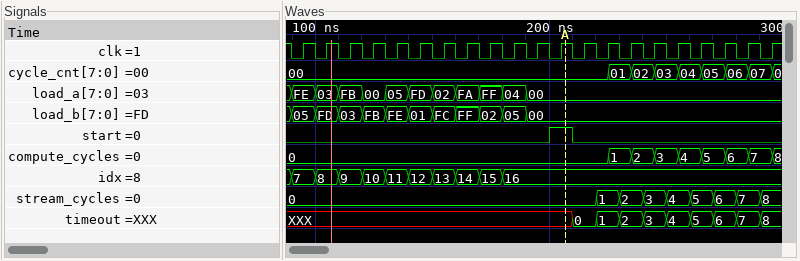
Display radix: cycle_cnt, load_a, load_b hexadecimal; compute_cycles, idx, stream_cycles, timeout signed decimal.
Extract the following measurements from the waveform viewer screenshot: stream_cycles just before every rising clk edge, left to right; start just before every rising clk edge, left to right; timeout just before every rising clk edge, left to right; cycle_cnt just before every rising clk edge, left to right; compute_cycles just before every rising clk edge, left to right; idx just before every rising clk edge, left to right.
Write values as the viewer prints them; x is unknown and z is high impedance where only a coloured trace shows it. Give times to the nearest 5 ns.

0, 0, 0, 0, 0, 0, 0, 0, 0, 0, 0, 0, 0, 1, 2, 3, 4, 5, 6, 7, 8
0 0 0 0 0 0 0 0 0 0 0 1 0 0 0 0 0 0 0 0 0
XXX, XXX, XXX, XXX, XXX, XXX, XXX, XXX, XXX, XXX, XXX, XXX, 0, 1, 2, 3, 4, 5, 6, 7, 8
00, 00, 00, 00, 00, 00, 00, 00, 00, 00, 00, 00, 00, 00, 01, 02, 03, 04, 05, 06, 07
0, 0, 0, 0, 0, 0, 0, 0, 0, 0, 0, 0, 0, 0, 1, 2, 3, 4, 5, 6, 7
7, 8, 9, 10, 11, 12, 13, 14, 15, 16, 16, 16, 16, 16, 16, 16, 16, 16, 16, 16, 16
